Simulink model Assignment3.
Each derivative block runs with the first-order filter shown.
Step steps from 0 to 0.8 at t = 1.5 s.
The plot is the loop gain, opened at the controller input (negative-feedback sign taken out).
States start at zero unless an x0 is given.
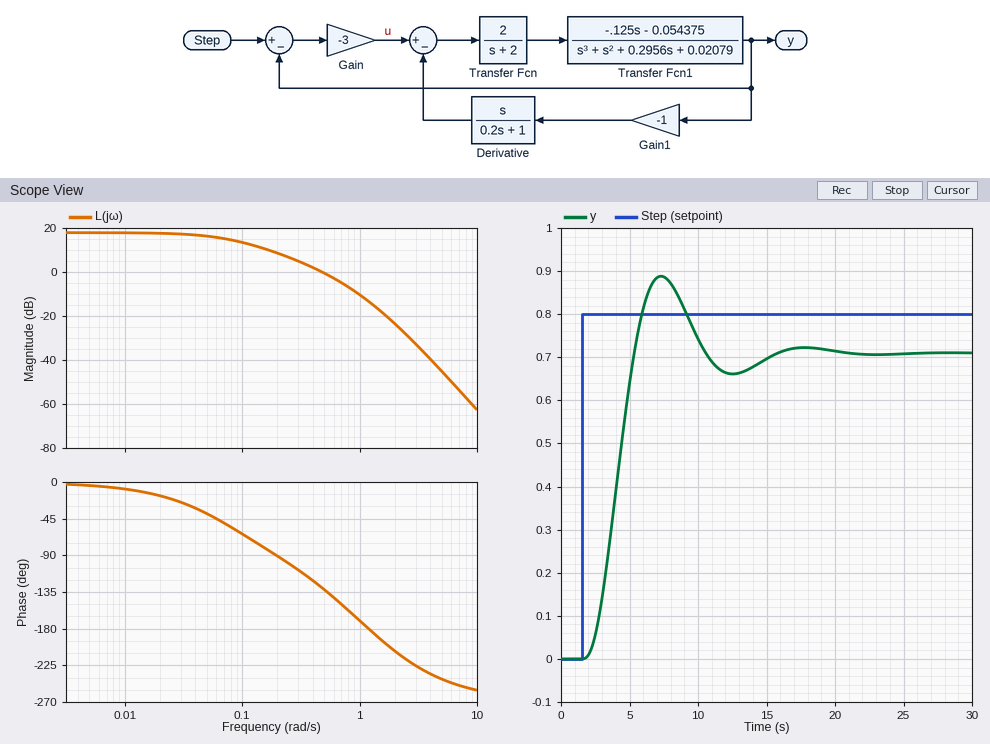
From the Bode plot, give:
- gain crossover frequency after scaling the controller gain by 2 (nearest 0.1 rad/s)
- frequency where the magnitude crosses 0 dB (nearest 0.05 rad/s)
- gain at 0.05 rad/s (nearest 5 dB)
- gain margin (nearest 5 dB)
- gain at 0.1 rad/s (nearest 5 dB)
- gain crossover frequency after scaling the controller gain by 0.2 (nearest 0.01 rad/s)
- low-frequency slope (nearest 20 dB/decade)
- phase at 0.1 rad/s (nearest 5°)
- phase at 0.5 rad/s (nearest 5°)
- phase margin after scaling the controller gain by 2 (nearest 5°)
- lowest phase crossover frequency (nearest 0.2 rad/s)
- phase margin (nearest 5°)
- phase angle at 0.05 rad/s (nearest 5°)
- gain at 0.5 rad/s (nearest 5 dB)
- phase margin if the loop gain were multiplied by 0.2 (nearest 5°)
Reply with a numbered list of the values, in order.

1. 0.8 rad/s
2. 0.50 rad/s
3. 15 dB
4. 15 dB
5. 15 dB
6. 0.09 rad/s
7. 0 dB/decade
8. -65°
9. -130°
10. 25°
11. 1.2 rad/s
12. 50°
13. -40°
14. 0 dB
15. 120°
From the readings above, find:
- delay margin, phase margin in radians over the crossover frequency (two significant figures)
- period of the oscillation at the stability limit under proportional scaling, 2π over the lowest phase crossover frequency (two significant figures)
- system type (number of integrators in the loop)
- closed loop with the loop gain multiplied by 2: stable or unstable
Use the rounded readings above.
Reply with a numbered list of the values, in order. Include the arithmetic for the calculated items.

1. 50 × π / 180 / 0.5 = 1.7 s
2. 2π / 1.2 = 5.2 s
3. 0
4. stable
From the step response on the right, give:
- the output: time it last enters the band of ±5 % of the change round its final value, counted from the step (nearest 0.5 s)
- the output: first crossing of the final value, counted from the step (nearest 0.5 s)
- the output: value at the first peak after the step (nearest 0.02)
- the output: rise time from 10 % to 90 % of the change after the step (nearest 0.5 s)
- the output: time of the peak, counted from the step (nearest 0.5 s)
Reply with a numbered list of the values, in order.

1. 12.5 s
2. 4.0 s
3. 0.88
4. 2.5 s
5. 6.0 s
